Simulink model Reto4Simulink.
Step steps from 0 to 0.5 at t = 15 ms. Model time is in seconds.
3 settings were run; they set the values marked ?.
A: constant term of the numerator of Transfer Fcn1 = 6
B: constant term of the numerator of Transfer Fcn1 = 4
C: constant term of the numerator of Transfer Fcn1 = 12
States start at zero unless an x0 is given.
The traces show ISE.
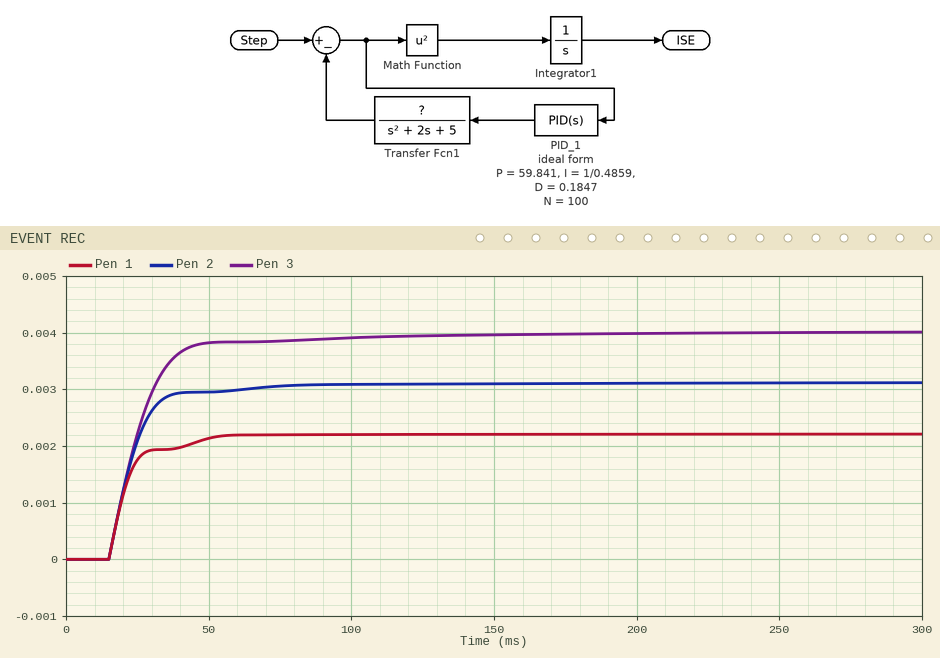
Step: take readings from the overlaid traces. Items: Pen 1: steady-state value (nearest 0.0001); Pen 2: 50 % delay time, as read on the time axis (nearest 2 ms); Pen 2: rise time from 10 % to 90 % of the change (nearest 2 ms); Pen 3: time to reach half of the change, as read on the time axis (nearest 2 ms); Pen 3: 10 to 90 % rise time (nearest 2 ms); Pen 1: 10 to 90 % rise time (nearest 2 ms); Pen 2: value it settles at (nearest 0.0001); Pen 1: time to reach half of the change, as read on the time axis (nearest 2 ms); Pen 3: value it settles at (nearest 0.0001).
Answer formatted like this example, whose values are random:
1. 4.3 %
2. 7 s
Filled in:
1. 0.0022
2. 22 ms
3. 18 ms
4. 24 ms
5. 22 ms
6. 26 ms
7. 0.0031
8. 20 ms
9. 0.0040
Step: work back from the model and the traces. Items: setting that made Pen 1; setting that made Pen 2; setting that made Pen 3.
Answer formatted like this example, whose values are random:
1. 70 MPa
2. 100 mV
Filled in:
1. C
2. A
3. B
